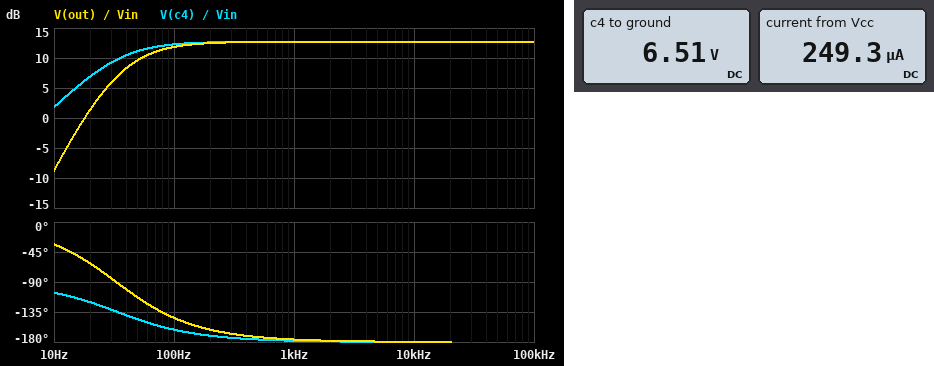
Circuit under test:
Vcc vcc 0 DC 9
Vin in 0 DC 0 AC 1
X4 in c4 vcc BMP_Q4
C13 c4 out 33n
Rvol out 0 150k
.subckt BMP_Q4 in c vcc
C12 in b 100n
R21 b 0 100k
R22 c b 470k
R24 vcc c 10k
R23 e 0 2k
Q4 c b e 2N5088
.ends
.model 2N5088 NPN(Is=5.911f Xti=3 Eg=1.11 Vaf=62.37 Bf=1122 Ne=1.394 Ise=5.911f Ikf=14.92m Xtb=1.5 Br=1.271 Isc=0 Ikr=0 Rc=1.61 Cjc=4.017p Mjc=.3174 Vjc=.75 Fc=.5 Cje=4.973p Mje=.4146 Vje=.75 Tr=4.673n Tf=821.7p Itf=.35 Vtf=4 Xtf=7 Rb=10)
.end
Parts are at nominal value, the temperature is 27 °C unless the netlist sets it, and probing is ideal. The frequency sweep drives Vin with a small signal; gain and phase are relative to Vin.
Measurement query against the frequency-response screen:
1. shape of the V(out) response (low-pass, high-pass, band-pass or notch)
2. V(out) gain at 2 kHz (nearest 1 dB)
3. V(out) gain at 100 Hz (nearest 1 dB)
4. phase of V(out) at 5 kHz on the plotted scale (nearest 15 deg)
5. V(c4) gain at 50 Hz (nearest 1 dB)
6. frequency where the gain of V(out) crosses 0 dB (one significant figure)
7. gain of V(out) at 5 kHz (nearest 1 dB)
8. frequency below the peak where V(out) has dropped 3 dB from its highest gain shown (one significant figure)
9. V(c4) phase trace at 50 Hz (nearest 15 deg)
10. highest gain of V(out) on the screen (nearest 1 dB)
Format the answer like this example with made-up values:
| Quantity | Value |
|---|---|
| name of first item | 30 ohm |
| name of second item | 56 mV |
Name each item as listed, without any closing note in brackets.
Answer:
| Quantity | Value |
|---|---|
| shape of the V(out) response | high-pass |
| V(out) gain at 2 kHz | 13 dB |
| V(out) gain at 100 Hz | 12 dB |
| phase of V(out) at 5 kHz on the plotted scale | -180 deg |
| V(c4) gain at 50 Hz | 11 dB |
| frequency where the gain of V(out) crosses 0 dB | 20 Hz |
| gain of V(out) at 5 kHz | 13 dB |
| frequency below the peak where V(out) has dropped 3 dB from its highest gain shown | 50 Hz |
| V(c4) phase trace at 50 Hz | -150 deg |
| highest gain of V(out) on the screen | 13 dB |
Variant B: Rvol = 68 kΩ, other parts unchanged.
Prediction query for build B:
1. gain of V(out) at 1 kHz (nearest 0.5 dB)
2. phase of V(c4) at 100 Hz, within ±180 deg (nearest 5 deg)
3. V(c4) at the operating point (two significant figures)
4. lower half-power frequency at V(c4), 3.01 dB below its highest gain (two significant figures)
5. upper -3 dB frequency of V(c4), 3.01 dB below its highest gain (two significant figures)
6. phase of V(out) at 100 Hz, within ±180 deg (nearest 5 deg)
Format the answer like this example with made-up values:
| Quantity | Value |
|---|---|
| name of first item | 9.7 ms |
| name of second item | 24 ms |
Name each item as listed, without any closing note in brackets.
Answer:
| Quantity | Value |
|---|---|
| gain of V(out) at 1 kHz | 12.0 dB |
| phase of V(c4) at 100 Hz, within ±180 deg | -165 deg |
| V(c4) at the operating point | 6.5 V |
| lower half-power frequency at V(c4), 3.01 dB below its highest gain | 29 Hz |
| upper -3 dB frequency of V(c4), 3.01 dB below its highest gain | 10 MHz |
| phase of V(out) at 100 Hz, within ±180 deg | -130 deg |
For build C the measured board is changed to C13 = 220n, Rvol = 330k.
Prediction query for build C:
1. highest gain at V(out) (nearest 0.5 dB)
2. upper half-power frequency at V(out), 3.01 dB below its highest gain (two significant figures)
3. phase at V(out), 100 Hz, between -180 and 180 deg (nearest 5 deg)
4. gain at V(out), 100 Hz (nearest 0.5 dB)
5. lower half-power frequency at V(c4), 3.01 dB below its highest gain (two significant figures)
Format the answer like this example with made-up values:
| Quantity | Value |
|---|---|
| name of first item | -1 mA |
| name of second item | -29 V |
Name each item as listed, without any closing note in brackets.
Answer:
| Quantity | Value |
|---|---|
| highest gain at V(out) | 13.0 dB |
| upper half-power frequency at V(out), 3.01 dB below its highest gain | 8.8 MHz |
| phase at V(out), 100 Hz, between -180 and 180 deg | -160 deg |
| gain at V(out), 100 Hz | 12.5 dB |
| lower half-power frequency at V(c4), 3.01 dB below its highest gain | 36 Hz |
